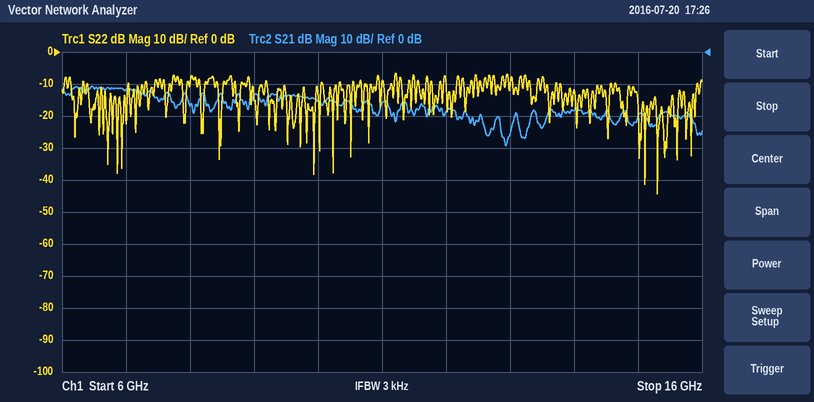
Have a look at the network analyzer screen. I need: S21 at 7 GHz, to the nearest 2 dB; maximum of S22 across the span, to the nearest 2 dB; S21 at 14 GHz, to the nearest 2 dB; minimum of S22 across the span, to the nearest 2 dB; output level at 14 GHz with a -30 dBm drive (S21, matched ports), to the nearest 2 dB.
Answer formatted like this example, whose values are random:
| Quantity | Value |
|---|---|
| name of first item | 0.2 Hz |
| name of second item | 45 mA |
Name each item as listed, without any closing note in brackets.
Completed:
| Quantity | Value |
|---|---|
| S21 at 7 GHz, to the nearest 2 dB | -12 dB |
| maximum of S22 across the span, to the nearest 2 dB | -6 dB |
| S21 at 14 GHz, to the nearest 2 dB | -18 dB |
| minimum of S22 across the span, to the nearest 2 dB | -44 dB |
| output level at 14 GHz with a -30 dBm drive (S21, matched ports), to the nearest 2 dB | -48 dBm |
